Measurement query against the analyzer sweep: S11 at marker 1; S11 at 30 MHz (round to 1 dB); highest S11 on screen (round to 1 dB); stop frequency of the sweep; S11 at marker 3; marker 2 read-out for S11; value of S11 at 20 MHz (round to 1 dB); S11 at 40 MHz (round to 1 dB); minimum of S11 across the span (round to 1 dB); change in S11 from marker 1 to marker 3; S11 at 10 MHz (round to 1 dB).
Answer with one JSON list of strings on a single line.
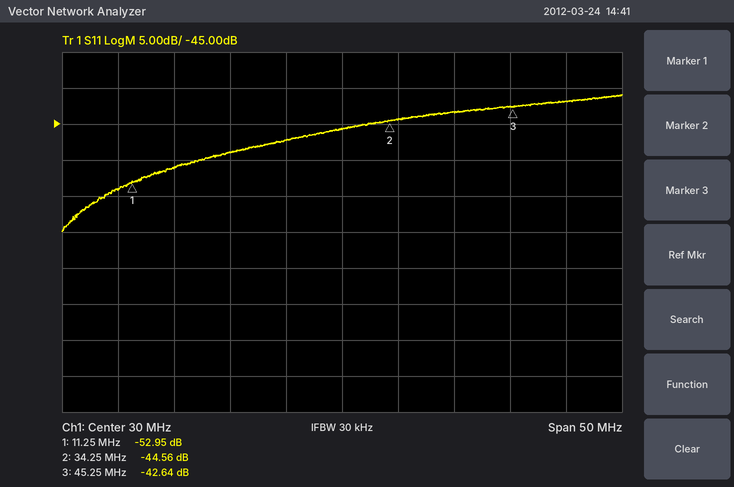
["-52.95 dB", "-46 dB", "-41 dB", "55 MHz", "-42.64 dB", "-44.56 dB", "-49 dB", "-43 dB", "-60 dB", "10.31 dB", "-54 dB"]
